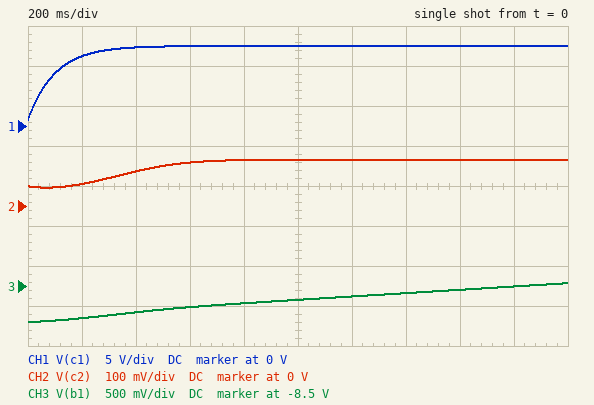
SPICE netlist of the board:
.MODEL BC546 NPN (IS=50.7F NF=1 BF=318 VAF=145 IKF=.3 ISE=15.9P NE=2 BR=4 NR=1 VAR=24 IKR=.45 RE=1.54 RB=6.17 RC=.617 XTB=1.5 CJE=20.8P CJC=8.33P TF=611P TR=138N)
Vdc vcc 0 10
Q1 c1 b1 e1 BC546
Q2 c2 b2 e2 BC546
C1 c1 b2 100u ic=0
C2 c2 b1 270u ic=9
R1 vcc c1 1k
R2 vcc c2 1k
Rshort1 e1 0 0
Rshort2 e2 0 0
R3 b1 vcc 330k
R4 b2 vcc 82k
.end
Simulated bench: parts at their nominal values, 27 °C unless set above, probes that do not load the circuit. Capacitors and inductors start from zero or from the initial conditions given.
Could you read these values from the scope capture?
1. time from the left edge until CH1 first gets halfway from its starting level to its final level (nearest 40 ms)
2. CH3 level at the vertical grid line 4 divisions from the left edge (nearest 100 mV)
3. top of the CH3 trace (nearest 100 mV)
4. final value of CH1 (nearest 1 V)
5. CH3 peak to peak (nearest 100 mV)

80 ms
-8.7 V
-8.5 V
10 V
500 mV
